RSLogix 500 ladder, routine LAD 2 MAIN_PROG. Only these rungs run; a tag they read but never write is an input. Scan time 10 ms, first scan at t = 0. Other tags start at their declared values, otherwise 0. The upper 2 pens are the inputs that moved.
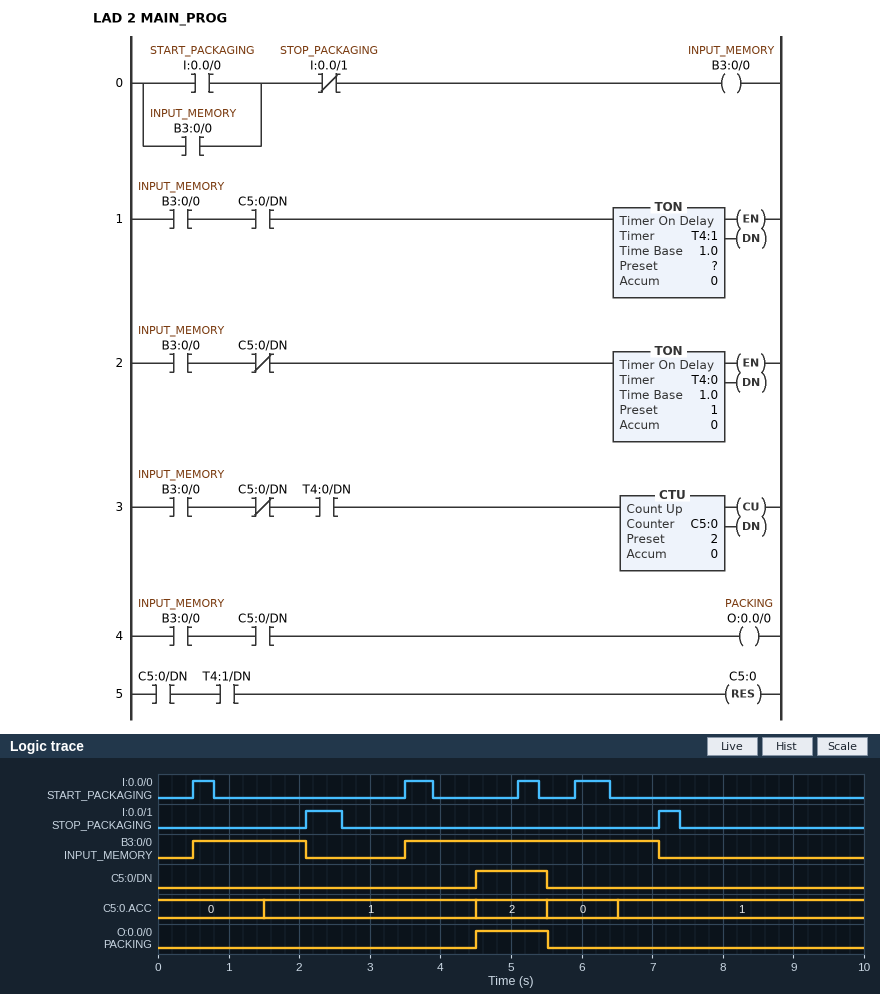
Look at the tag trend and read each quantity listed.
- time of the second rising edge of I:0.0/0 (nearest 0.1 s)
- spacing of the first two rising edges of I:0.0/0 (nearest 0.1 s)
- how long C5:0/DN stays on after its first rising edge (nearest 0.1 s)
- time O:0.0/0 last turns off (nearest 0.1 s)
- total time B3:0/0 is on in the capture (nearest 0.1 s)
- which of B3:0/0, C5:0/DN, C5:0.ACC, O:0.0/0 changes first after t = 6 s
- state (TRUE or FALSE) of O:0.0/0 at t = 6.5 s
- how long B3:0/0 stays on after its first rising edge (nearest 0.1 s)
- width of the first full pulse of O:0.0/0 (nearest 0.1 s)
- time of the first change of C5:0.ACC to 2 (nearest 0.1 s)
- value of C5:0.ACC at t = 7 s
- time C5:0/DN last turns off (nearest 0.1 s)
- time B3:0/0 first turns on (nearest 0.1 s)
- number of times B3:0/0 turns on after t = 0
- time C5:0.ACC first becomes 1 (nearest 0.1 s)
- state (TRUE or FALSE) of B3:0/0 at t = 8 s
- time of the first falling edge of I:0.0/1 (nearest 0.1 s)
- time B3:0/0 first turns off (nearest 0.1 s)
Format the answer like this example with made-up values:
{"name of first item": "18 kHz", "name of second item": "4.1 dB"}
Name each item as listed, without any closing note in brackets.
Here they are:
{"time of the second rising edge of I:0.0/0": "3.5 s", "spacing of the first two rising edges of I:0.0/0": "3.0 s", "how long C5:0/DN stays on after its first rising edge": "1.0 s", "time O:0.0/0 last turns off": "5.5 s", "total time B3:0/0 is on in the capture": "5.2 s", "which of B3:0/0, C5:0/DN, C5:0.ACC, O:0.0/0 changes first after t = 6 s": "C5:0.ACC", "state (TRUE or FALSE) of O:0.0/0 at t = 6.5 s": "FALSE", "how long B3:0/0 stays on after its first rising edge": "1.6 s", "width of the first full pulse of O:0.0/0": "1.0 s", "time of the first change of C5:0.ACC to 2": "4.5 s", "value of C5:0.ACC at t = 7 s": "1", "time C5:0/DN last turns off": "5.5 s", "time B3:0/0 first turns on": "0.5 s", "number of times B3:0/0 turns on after t = 0": "2", "time C5:0.ACC first becomes 1": "1.5 s", "state (TRUE or FALSE) of B3:0/0 at t = 8 s": "FALSE", "time of the first falling edge of I:0.0/1": "2.6 s", "time B3:0/0 first turns off": "2.1 s"}
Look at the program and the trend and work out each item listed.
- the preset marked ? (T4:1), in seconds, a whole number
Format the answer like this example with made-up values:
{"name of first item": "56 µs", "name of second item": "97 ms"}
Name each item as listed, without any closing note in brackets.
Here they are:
{"the preset marked ? (T4:1), in seconds, a whole number": "1 s"}
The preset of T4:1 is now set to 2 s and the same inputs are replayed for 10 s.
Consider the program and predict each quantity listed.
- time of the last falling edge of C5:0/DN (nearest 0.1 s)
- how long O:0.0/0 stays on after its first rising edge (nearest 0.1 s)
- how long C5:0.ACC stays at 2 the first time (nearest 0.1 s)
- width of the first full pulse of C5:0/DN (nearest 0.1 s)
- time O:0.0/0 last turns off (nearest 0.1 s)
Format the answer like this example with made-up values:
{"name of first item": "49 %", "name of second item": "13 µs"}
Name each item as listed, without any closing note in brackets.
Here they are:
{"time of the last falling edge of C5:0/DN": "6.5 s", "how long O:0.0/0 stays on after its first rising edge": "2.0 s", "how long C5:0.ACC stays at 2 the first time": "2.0 s", "width of the first full pulse of C5:0/DN": "2.0 s", "time O:0.0/0 last turns off": "6.5 s"}
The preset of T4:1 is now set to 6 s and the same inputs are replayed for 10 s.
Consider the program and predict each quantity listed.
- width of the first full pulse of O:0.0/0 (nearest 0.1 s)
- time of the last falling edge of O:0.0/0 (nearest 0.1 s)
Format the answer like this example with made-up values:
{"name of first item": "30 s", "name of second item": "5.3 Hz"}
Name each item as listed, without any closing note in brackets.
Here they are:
{"width of the first full pulse of O:0.0/0": "2.6 s", "time of the last falling edge of O:0.0/0": "7.1 s"}
